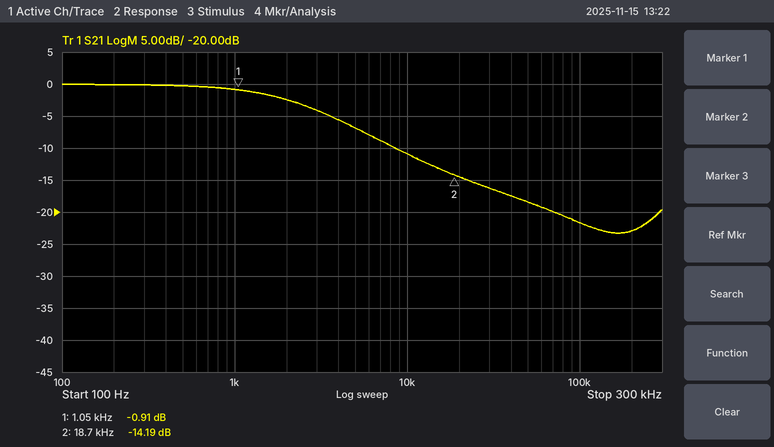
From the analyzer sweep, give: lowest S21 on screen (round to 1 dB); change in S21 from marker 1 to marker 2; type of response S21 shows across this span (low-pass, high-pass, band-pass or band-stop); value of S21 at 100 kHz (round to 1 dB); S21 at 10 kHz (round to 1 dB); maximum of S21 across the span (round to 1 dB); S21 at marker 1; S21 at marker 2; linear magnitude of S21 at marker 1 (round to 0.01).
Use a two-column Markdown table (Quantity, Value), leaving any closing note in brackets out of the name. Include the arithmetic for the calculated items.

| Quantity | Value |
|---|---|
| lowest S21 on screen | -23 dB |
| change in S21 from marker 1 to marker 2 | -14.19 − (-0.91) = -13.28 dB |
| type of response S21 shows across this span | low-pass |
| value of S21 at 100 kHz | -22 dB |
| S21 at 10 kHz | -11 dB |
| maximum of S21 across the span | 0 dB |
| S21 at marker 1 | -0.91 dB |
| S21 at marker 2 | -14.19 dB |
| linear magnitude of S21 at marker 1 | 10^(-0.91/20) ≈ 0.90 |
